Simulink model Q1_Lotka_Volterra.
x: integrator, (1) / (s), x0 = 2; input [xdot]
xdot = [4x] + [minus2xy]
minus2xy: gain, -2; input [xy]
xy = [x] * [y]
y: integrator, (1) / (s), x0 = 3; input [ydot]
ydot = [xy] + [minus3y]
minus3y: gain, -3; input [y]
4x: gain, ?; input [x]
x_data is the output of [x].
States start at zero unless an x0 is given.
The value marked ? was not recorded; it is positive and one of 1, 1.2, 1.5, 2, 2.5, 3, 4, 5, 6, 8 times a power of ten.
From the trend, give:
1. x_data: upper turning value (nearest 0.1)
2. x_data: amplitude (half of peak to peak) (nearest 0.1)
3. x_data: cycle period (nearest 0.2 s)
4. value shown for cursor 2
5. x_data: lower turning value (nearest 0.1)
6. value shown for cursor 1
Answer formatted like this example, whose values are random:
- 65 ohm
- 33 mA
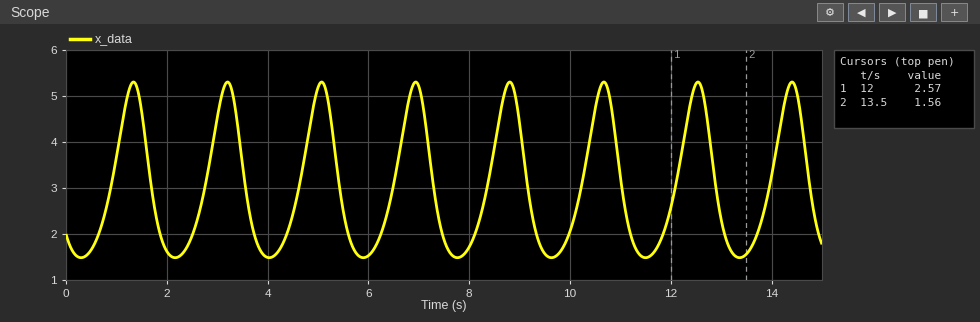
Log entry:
- 5.3
- 1.9
- 1.8 s
- 1.56
- 1.5
- 2.57
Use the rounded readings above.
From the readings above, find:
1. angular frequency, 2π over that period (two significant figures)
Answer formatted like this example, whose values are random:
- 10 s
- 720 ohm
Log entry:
- 3.5 rad/s
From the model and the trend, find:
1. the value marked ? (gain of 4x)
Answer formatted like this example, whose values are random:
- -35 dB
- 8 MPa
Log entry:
- 4
